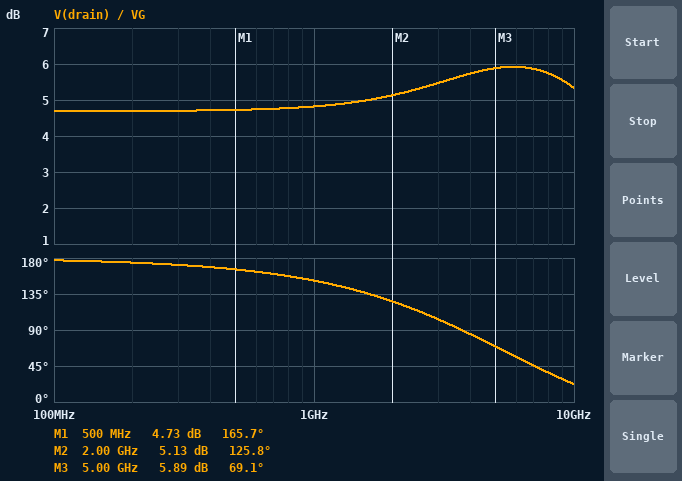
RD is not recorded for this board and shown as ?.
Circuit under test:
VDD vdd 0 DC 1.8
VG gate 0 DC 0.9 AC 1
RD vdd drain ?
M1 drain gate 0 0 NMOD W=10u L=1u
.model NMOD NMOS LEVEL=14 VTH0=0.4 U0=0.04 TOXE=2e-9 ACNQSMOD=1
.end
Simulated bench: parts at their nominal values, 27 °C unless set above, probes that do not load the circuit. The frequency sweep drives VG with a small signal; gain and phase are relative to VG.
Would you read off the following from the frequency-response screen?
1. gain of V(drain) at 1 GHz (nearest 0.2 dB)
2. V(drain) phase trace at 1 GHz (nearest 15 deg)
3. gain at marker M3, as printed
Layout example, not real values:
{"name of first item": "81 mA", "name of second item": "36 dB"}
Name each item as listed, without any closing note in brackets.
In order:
{"gain of V(drain) at 1 GHz": "4.8 dB", "V(drain) phase trace at 1 GHz": "150 deg", "gain at marker M3, as printed": "5.89 dB"}
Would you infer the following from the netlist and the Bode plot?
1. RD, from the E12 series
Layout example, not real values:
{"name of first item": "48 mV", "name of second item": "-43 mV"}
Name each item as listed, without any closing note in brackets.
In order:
{"RD, from the E12 series": "1.2 kΩ"}
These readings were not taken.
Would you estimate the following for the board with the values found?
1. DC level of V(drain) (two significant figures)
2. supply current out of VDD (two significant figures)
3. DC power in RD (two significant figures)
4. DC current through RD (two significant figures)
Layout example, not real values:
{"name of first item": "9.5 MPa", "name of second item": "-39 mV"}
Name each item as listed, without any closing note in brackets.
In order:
{"DC level of V(drain)": "1.3 V", "supply current out of VDD": "420 µA", "DC power in RD": "210 µW", "DC current through RD": "420 µA"}
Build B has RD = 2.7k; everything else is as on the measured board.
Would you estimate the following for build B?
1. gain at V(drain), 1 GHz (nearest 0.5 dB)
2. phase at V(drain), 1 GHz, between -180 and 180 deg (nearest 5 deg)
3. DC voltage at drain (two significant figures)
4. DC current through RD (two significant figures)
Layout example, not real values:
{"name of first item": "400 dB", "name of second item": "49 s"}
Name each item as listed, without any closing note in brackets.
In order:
{"gain at V(drain), 1 GHz": "10.5 dB", "phase at V(drain), 1 GHz, between -180 and 180 deg": "140 deg", "DC voltage at drain": "720 mV", "DC current through RD": "400 µA"}
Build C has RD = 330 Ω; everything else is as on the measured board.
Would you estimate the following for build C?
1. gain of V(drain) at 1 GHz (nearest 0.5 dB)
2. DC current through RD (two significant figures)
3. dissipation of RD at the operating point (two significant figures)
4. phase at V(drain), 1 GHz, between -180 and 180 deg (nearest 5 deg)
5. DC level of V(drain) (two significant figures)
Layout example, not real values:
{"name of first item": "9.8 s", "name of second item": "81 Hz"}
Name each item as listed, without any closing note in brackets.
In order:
{"gain of V(drain) at 1 GHz": "-6.0 dB", "DC current through RD": "430 µA", "dissipation of RD at the operating point": "61 µW", "phase at V(drain), 1 GHz, between -180 and 180 deg": "160 deg", "DC level of V(drain)": "1.7 V"}
